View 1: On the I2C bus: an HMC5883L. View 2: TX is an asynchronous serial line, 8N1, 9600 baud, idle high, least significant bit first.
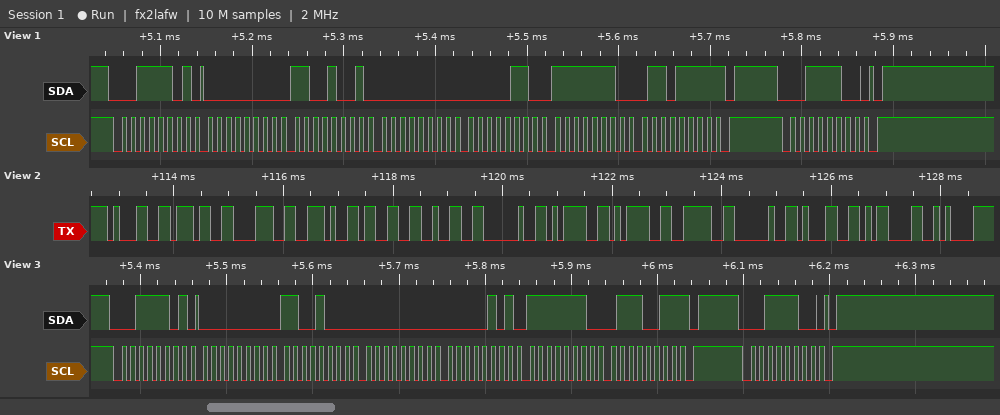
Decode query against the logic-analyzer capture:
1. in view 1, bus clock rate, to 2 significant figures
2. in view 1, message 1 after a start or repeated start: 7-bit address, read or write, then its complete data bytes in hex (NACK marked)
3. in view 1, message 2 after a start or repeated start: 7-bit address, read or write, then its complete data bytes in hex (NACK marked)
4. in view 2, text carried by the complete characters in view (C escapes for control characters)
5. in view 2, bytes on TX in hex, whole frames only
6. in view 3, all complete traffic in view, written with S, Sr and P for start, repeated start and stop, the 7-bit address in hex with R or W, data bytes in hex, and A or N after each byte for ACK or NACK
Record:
100 kHz
0x1E read: 00 C9 00 06 FE 6F NACK
0x1E write
"178.32 ==> 1\r\n"
31 37 38 2E 33 32 20 3D 3D 3E 20 31 0D 0A
S 1ER A 00 A C8 A 00 A 05 A FE A 73 N P S 1EW A P
